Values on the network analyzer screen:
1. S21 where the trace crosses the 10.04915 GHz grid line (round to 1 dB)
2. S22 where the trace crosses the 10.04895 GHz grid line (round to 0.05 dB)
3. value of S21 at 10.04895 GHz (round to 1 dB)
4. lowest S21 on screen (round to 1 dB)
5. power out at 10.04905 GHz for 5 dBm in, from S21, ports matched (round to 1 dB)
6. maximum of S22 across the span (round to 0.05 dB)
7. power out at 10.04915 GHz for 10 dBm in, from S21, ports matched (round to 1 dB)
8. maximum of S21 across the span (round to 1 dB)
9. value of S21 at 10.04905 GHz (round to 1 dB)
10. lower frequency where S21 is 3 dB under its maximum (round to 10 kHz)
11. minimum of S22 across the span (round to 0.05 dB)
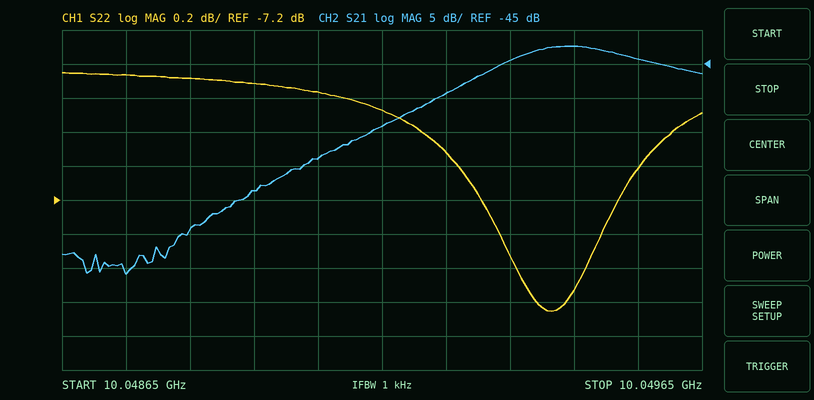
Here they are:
-54 dB
-6.50 dB
-64 dB
-76 dB
-54 dBm
-6.45 dB
-44 dBm
-42 dB
-59 dB
10.04933 GHz
-7.85 dB
